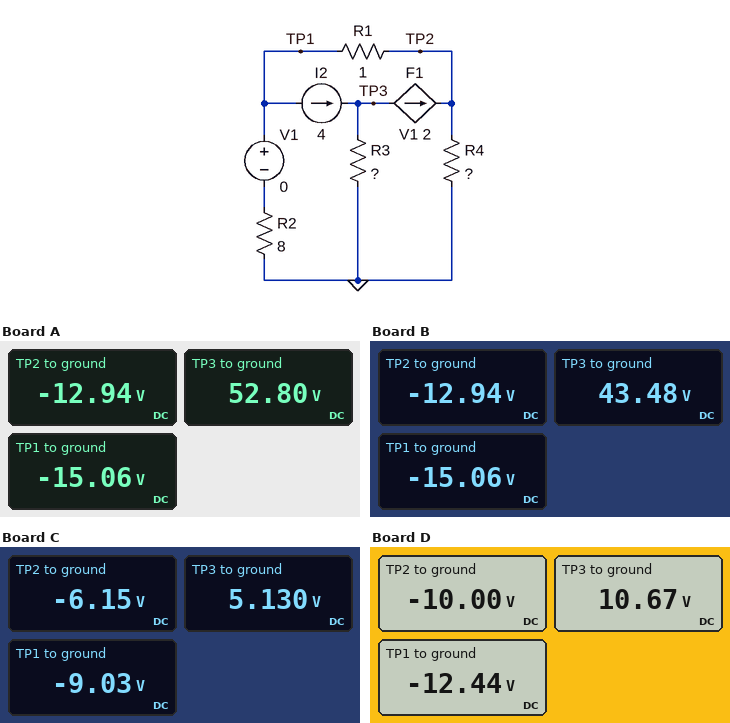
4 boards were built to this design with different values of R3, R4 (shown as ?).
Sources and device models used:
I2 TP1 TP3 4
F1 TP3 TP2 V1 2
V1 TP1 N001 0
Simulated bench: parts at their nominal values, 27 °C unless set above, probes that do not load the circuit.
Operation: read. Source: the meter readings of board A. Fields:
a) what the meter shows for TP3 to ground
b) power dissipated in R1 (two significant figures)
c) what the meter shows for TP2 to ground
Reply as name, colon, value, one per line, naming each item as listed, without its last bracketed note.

what the meter shows for TP3 to ground: 52.80 V
power dissipated in R1: 4.5 W
what the meter shows for TP2 to ground: -12.94 V
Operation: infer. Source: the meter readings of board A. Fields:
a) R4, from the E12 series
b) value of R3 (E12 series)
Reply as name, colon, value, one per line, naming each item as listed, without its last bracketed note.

R4, from the E12 series: 2.2 Ω
value of R3: 6.8 Ω
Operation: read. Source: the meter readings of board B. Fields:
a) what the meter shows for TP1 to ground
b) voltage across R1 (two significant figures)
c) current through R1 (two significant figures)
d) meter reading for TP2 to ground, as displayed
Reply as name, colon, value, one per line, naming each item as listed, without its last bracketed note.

what the meter shows for TP1 to ground: -15.06 V
voltage across R1: 2.1 V
current through R1: 2.1 A
meter reading for TP2 to ground, as displayed: -12.94 V
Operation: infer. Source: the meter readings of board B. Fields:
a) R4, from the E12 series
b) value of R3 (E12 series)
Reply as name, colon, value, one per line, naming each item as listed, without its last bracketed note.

R4, from the E12 series: 2.2 Ω
value of R3: 5.6 Ω
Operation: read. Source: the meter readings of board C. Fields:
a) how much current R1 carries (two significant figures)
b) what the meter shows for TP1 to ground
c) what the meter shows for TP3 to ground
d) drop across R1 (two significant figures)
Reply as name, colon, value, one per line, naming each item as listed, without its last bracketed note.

how much current R1 carries: 2.9 A
what the meter shows for TP1 to ground: -9.03 V
what the meter shows for TP3 to ground: 5.130 V
drop across R1: 2.9 V
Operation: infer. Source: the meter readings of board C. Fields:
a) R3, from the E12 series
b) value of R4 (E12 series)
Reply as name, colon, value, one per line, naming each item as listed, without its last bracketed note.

R3, from the E12 series: 0.82 Ω
value of R4: 1.2 Ω
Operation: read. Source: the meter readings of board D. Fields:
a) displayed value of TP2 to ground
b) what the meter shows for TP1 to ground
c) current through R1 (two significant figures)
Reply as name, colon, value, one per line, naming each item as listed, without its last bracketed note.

displayed value of TP2 to ground: -10.00 V
what the meter shows for TP1 to ground: -12.44 V
current through R1: 2.4 A
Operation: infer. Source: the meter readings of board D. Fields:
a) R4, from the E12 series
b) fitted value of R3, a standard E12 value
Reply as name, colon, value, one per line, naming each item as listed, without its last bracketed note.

R4, from the E12 series: 1.8 Ω
fitted value of R3, a standard E12 value: 1.5 Ω
